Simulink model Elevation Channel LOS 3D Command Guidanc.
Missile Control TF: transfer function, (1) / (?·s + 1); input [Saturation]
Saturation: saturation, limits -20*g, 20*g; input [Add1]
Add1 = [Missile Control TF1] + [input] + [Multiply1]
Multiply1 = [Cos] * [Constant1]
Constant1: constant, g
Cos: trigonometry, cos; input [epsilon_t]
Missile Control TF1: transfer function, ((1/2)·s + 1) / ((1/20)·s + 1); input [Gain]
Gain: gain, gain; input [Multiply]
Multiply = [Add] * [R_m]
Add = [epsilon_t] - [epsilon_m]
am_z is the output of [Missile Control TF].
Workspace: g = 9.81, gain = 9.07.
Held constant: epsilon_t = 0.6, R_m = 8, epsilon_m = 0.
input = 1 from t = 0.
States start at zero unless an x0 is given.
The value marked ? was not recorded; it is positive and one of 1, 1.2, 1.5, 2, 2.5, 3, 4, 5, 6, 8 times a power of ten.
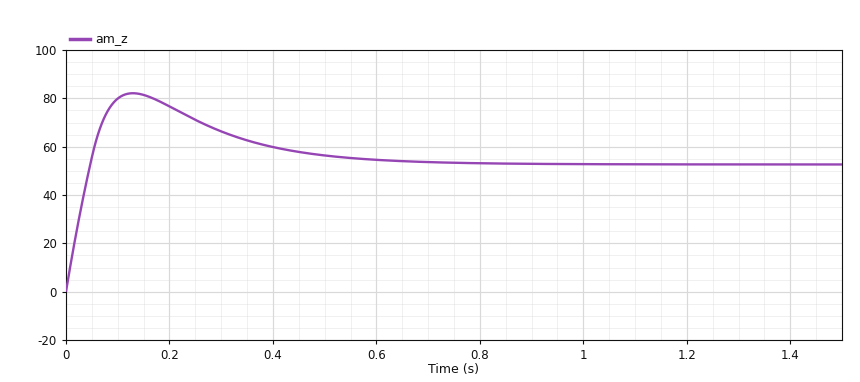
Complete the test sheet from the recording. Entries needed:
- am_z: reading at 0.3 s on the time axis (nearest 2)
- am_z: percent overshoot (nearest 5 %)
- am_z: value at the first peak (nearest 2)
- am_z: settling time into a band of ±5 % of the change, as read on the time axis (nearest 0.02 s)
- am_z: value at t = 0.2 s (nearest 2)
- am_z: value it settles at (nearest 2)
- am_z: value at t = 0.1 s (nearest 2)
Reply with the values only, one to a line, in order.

66
55 %
82
0.56 s
76
52
80
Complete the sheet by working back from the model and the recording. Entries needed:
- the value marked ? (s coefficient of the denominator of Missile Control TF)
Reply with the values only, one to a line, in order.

0.15
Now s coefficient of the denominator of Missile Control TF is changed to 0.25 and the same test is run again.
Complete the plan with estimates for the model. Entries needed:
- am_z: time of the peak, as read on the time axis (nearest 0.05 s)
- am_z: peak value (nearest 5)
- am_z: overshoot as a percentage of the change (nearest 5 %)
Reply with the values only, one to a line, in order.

0.20 s
60
15 %
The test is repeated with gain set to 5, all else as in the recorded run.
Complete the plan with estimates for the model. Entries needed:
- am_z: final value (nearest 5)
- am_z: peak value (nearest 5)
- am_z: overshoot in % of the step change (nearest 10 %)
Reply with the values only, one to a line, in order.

35
55
70 %
